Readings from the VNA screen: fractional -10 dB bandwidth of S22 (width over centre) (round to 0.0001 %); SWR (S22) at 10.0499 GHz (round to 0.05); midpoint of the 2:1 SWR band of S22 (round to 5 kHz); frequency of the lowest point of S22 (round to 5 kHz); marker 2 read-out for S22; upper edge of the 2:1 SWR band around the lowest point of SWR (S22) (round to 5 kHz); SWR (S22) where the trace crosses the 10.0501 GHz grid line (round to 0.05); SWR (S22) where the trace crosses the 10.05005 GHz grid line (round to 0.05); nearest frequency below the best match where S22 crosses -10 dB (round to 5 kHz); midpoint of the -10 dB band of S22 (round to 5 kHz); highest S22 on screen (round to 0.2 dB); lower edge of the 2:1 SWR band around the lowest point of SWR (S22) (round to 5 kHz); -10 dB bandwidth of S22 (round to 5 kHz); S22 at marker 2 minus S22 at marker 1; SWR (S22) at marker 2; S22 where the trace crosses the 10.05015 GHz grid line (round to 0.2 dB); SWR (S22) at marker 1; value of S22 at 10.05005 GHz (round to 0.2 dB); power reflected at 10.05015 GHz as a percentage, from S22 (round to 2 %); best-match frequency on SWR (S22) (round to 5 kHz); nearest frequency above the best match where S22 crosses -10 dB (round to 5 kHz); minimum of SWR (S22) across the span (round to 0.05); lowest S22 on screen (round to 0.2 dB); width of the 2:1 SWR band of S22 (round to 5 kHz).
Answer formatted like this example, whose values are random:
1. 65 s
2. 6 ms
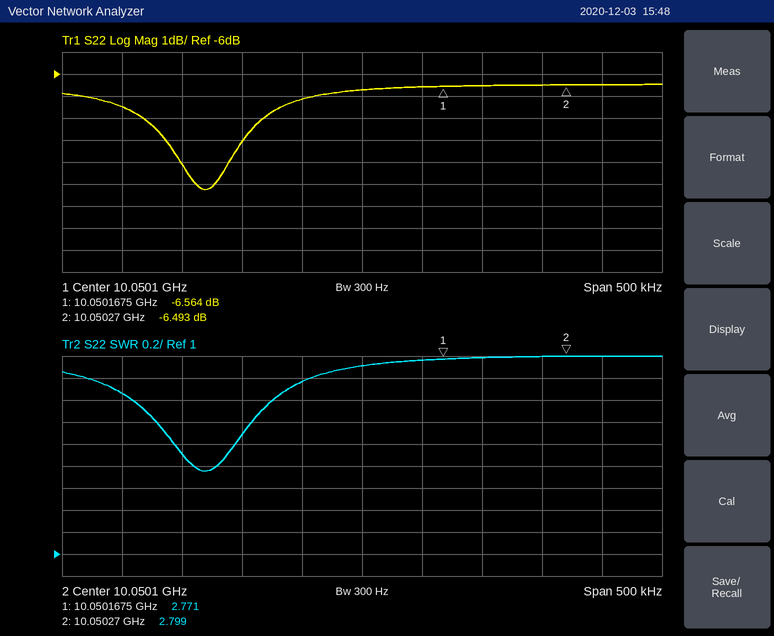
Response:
1. 0.0004 %
2. 2.45
3. 10.049970 GHz
4. 10.049970 GHz
5. -6.493 dB
6. 10.049995 GHz
7. 2.70
8. 2.55
9. 10.049950 GHz
10. 10.049970 GHz
11. -6.4 dB
12. 10.049945 GHz
13. 40 kHz
14. 0.071 dB
15. 2.799
16. -6.6 dB
17. 2.771
18. -7.2 dB
19. 22 %
20. 10.049970 GHz
21. 10.049990 GHz
22. 1.75
23. -11.2 dB
24. 50 kHz
